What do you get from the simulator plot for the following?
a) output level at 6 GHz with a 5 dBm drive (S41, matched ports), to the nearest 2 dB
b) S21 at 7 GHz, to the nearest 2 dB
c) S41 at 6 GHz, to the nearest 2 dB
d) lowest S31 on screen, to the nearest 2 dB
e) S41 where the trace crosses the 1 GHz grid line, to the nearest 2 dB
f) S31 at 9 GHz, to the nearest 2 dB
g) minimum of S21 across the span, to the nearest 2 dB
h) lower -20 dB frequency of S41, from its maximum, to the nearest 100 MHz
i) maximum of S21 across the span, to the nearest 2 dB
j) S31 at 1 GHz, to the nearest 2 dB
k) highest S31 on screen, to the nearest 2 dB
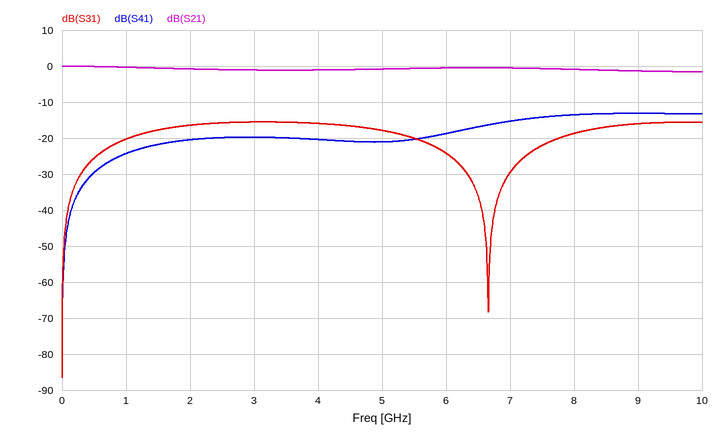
-14 dBm
0 dB
-18 dB
-86 dB
-24 dB
-16 dB
-2 dB
300 MHz
0 dB
-20 dB
-16 dB
